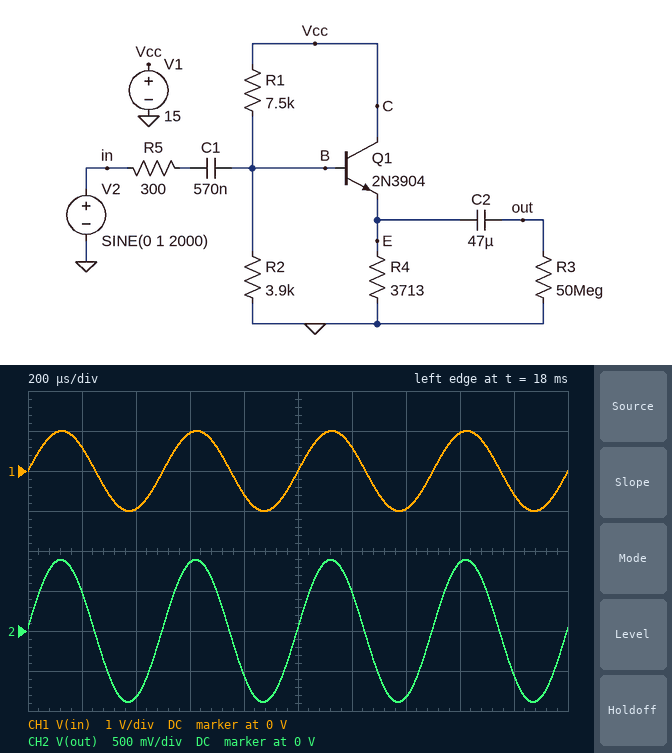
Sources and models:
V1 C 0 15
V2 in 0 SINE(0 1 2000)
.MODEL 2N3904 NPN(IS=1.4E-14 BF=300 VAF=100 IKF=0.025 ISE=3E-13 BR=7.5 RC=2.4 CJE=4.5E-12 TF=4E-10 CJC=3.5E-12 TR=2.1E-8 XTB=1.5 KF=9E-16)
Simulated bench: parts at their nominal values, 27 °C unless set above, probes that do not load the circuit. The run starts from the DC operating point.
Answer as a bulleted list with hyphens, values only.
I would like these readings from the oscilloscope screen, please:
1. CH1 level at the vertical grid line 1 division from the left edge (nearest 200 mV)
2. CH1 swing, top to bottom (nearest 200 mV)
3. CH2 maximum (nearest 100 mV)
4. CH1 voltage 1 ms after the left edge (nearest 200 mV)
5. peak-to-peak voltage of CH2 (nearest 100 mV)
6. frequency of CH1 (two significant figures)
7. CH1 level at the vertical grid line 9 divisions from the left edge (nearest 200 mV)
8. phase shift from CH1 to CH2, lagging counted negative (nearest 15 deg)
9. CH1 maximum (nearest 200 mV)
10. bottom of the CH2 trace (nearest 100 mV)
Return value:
- 600 mV
- 2.0 V
- 900 mV
- 0 V
- 1.8 V
- 2.0 kHz
- -600 mV
- 0 deg
- 1.0 V
- -900 mV
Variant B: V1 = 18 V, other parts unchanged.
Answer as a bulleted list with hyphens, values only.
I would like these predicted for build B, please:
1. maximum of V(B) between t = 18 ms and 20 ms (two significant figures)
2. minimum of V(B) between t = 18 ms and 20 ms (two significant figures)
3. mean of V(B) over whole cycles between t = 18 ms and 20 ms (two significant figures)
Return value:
- 7.0 V
- 5.2 V
- 6.1 V
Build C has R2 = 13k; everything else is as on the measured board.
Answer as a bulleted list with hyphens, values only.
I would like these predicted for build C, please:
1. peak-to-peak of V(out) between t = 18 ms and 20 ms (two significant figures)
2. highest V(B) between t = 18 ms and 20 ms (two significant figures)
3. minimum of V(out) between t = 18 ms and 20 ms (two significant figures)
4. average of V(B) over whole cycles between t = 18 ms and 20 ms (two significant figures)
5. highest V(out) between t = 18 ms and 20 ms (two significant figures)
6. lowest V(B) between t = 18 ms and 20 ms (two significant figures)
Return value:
- 1.9 V
- 10 V
- -940 mV
- 9.4 V
- 940 mV
- 8.5 V
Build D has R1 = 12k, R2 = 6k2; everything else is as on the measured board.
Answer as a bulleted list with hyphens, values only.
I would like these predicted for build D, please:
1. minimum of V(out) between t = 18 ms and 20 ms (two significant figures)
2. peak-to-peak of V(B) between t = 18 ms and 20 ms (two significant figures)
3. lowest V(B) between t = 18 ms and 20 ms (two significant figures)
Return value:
- -920 mV
- 1.9 V
- 4.1 V
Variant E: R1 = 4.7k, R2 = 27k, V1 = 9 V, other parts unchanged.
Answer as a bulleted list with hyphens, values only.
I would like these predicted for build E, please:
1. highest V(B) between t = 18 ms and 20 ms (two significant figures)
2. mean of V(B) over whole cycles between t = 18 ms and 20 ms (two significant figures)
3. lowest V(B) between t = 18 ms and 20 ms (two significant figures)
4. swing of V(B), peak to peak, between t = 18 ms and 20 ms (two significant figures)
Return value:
- 8.5 V
- 7.6 V
- 6.7 V
- 1.9 V
